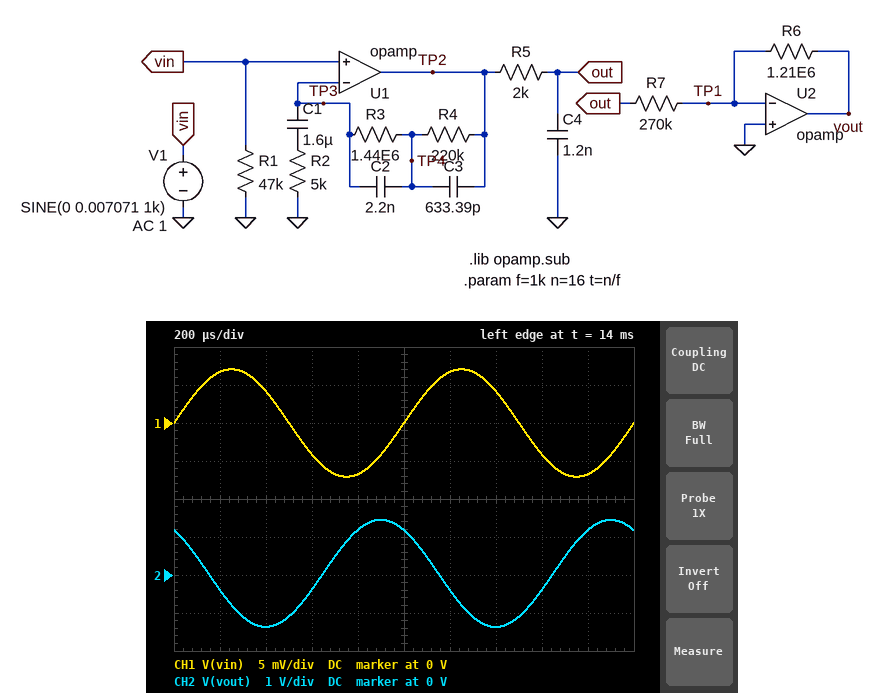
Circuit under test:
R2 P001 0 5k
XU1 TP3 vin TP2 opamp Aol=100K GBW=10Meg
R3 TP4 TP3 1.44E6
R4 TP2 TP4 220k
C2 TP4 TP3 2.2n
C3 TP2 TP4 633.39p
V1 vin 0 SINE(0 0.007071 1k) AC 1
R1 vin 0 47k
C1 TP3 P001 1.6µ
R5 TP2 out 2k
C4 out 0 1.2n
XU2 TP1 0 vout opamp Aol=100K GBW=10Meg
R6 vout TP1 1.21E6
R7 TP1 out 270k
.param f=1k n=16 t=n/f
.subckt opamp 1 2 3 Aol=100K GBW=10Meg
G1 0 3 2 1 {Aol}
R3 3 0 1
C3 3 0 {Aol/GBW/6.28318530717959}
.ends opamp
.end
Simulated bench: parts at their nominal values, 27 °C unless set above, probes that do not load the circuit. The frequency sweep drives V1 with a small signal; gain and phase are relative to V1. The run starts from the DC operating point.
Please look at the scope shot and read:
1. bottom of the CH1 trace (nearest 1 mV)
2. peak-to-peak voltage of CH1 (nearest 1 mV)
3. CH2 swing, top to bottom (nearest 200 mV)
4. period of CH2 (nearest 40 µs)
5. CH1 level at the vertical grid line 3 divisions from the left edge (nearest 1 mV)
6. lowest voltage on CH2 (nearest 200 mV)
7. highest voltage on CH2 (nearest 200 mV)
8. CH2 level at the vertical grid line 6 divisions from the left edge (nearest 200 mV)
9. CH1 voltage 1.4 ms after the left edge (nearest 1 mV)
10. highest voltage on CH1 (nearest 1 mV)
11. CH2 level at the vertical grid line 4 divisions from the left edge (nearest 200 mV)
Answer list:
-7 mV
14 mV
2.8 V
1.00 ms
-4 mV
-1.4 V
1.4 V
-400 mV
4 mV
7 mV
1.2 V
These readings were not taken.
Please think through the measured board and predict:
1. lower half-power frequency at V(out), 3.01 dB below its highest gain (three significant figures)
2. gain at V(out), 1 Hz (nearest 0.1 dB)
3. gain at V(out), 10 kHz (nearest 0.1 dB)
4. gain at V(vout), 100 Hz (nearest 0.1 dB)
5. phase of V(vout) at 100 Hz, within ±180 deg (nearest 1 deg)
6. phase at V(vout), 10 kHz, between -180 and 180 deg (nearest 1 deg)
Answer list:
12.2 Hz
24.4 dB
16.2 dB
56.7 dB
142 deg
95 deg
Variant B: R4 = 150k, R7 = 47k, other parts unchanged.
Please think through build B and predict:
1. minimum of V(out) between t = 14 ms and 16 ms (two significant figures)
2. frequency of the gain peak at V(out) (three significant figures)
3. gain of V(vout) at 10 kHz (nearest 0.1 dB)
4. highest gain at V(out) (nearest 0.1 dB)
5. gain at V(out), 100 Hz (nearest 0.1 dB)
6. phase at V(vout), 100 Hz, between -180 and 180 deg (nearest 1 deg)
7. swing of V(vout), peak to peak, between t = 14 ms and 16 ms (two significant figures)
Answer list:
-260 mV
31.8 Hz
44.1 dB
46.8 dB
42.8 dB
138 deg
13 V
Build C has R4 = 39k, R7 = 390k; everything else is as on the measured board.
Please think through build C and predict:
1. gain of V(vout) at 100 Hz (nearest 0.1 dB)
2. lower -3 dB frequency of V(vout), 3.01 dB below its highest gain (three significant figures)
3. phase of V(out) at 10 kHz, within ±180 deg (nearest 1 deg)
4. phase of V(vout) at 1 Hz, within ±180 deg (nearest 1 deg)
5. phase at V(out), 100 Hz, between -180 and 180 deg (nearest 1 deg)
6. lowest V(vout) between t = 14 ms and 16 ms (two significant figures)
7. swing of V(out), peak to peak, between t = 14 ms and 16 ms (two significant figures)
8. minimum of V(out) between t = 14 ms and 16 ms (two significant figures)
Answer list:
52.1 dB
12.1 Hz
-65 deg
-98 deg
-49 deg
-370 mV
260 mV
-140 mV
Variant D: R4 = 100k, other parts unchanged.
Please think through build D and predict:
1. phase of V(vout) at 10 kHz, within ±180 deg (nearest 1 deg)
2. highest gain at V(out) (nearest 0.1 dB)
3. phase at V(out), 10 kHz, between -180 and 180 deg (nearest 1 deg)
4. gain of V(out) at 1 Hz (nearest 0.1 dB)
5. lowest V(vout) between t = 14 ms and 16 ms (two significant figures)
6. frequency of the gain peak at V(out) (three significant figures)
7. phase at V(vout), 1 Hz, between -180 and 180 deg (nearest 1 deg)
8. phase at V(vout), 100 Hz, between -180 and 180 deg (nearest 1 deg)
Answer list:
101 deg
46.8 dB
-79 deg
23.8 dB
-860 mV
31.7 Hz
-98 deg
135 deg
